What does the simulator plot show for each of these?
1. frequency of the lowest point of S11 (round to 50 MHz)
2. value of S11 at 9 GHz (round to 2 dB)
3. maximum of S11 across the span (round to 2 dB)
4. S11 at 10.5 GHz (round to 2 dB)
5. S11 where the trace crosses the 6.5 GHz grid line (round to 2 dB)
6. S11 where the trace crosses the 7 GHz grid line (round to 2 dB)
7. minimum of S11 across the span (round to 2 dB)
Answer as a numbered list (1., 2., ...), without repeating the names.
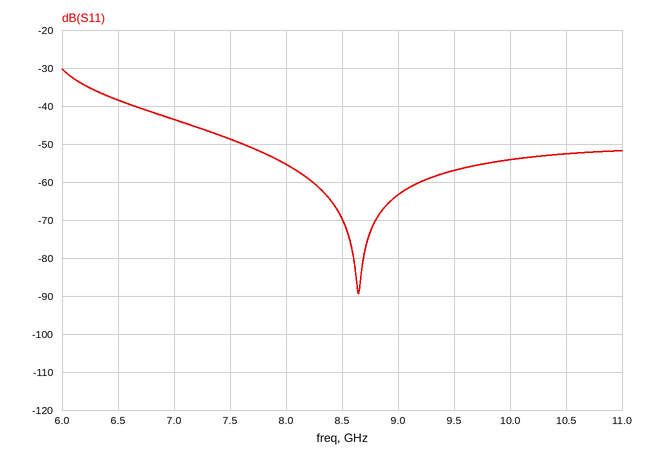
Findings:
1. 8.65 GHz
2. -64 dB
3. -30 dB
4. -52 dB
5. -38 dB
6. -44 dB
7. -90 dB
